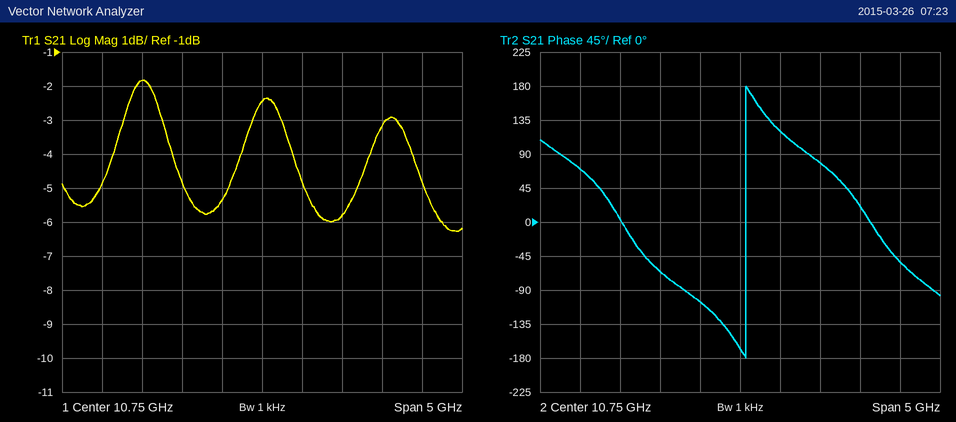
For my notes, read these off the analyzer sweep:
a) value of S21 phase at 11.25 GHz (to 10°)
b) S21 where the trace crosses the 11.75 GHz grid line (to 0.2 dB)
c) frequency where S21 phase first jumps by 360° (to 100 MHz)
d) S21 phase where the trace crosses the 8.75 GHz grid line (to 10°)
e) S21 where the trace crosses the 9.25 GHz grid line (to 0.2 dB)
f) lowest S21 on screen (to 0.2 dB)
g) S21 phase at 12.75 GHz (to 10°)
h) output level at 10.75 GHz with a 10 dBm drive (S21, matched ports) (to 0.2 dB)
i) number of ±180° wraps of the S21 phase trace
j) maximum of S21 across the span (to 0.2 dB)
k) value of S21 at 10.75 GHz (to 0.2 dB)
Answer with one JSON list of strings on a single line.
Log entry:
["120°", "-5.8 dB", "10.8 GHz", "70°", "-1.8 dB", "-6.2 dB", "-50°", "7.6 dBm", "1", "-1.8 dB", "-2.4 dB"]
